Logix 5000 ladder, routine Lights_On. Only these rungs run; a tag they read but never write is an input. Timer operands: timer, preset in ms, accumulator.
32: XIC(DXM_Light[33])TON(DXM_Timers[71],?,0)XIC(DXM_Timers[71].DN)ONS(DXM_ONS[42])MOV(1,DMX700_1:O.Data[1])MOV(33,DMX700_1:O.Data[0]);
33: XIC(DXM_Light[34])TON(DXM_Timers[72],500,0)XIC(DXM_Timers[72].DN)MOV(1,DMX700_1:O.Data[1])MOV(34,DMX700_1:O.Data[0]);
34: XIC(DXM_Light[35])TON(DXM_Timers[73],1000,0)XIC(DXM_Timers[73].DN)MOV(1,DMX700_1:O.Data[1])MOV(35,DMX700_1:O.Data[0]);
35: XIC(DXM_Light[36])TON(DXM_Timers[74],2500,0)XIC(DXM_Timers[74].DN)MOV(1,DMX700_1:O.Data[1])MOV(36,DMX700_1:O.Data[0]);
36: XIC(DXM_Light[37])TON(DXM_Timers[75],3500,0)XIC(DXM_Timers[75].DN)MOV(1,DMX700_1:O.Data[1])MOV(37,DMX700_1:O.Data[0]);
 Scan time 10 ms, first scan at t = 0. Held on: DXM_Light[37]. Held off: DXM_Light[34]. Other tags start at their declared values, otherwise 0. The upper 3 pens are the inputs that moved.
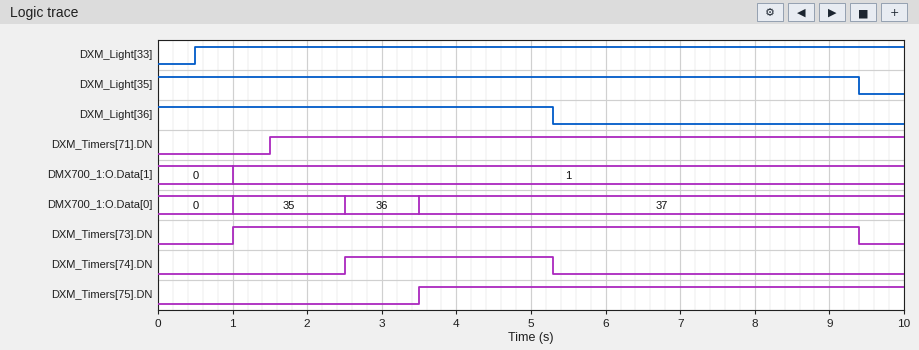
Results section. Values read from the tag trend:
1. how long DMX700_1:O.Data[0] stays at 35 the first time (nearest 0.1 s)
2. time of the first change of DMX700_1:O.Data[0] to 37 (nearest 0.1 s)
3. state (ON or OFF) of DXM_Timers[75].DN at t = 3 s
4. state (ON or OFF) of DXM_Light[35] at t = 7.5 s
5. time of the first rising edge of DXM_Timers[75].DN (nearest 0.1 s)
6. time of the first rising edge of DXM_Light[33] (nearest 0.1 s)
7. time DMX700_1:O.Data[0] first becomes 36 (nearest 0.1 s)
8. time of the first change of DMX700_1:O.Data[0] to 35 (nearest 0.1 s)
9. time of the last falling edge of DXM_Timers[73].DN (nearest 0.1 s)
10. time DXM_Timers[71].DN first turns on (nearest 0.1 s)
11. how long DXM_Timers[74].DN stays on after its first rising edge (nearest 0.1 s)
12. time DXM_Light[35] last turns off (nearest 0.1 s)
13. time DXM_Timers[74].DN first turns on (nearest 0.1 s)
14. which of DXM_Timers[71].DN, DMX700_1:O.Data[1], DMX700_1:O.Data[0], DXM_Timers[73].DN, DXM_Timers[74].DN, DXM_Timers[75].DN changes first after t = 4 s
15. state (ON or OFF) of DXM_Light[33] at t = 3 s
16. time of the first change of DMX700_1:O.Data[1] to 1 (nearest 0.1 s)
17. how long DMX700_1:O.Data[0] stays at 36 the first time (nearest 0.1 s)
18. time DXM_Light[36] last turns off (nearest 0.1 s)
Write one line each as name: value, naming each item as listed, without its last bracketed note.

how long DMX700_1:O.Data[0] stays at 35 the first time: 1.5 s
time of the first change of DMX700_1:O.Data[0] to 37: 3.5 s
state (ON or OFF) of DXM_Timers[75].DN at t = 3 s: OFF
state (ON or OFF) of DXM_Light[35] at t = 7.5 s: ON
time of the first rising edge of DXM_Timers[75].DN: 3.5 s
time of the first rising edge of DXM_Light[33]: 0.5 s
time DMX700_1:O.Data[0] first becomes 36: 2.5 s
time of the first change of DMX700_1:O.Data[0] to 35: 1.0 s
time of the last falling edge of DXM_Timers[73].DN: 9.4 s
time DXM_Timers[71].DN first turns on: 1.5 s
how long DXM_Timers[74].DN stays on after its first rising edge: 2.8 s
time DXM_Light[35] last turns off: 9.4 s
time DXM_Timers[74].DN first turns on: 2.5 s
which of DXM_Timers[71].DN, DMX700_1:O.Data[1], DMX700_1:O.Data[0], DXM_Timers[73].DN, DXM_Timers[74].DN, DXM_Timers[75].DN changes first after t = 4 s: DXM_Timers[74].DN
state (ON or OFF) of DXM_Light[33] at t = 3 s: ON
time of the first change of DMX700_1:O.Data[1] to 1: 1.0 s
how long DMX700_1:O.Data[0] stays at 36 the first time: 1.0 s
time DXM_Light[36] last turns off: 5.3 s
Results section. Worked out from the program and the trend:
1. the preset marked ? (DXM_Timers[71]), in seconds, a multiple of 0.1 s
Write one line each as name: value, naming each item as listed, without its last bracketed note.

the preset marked ? (DXM_Timers[71]), in seconds, a multiple of 0.1 s: 1.0 s
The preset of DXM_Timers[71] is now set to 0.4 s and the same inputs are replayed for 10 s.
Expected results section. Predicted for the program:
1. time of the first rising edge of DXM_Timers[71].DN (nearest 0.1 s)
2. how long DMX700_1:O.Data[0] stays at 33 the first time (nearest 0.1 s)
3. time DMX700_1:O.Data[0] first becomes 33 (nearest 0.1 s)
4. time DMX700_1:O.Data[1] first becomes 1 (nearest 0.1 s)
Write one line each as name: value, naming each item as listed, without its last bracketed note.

time of the first rising edge of DXM_Timers[71].DN: 0.9 s
how long DMX700_1:O.Data[0] stays at 33 the first time: 0.1 s
time DMX700_1:O.Data[0] first becomes 33: 0.9 s
time DMX700_1:O.Data[1] first becomes 1: 0.9 s
